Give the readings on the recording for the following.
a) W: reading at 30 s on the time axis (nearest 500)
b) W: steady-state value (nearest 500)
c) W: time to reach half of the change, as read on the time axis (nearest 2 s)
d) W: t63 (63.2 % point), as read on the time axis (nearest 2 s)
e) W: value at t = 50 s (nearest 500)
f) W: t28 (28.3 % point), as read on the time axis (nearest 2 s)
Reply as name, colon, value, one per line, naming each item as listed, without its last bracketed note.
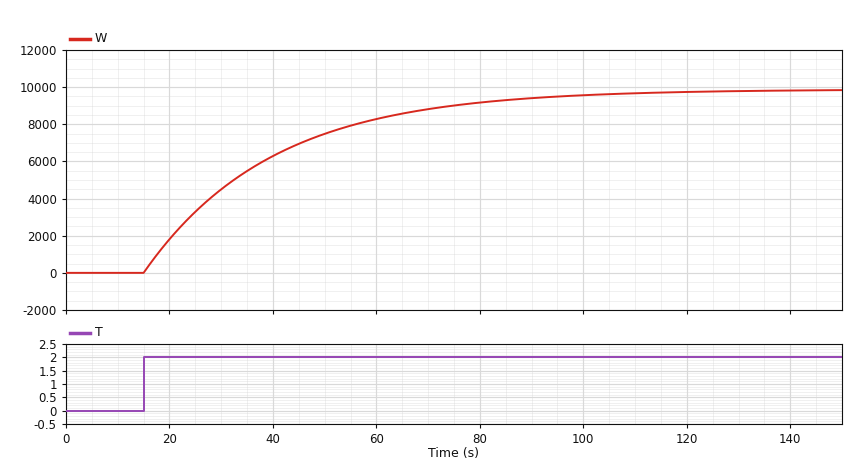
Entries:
W: reading at 30 s on the time axis: 4500
W: steady-state value: 10000
W: time to reach half of the change, as read on the time axis: 32 s
W: t63 (63.2 % point), as read on the time axis: 40 s
W: value at t = 50 s: 7500
W: t28 (28.3 % point), as read on the time axis: 24 s
